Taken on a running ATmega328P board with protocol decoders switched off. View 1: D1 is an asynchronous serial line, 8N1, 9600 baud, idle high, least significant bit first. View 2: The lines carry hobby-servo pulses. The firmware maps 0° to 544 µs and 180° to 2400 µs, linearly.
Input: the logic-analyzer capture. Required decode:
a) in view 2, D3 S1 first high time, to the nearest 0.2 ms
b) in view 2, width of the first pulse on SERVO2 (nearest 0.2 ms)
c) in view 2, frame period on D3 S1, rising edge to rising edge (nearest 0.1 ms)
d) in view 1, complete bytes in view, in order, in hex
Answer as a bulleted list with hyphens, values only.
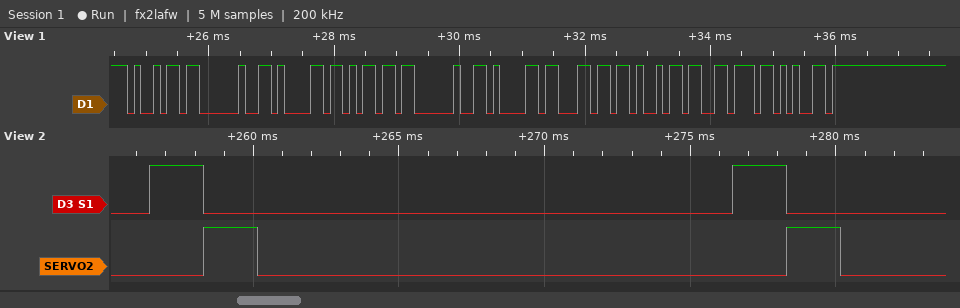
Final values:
- 1.8 ms
- 1.8 ms
- 20.0 ms
- 0x69 0x20 0x61 0x6D 0x20 0x61 0x6C 0x69 0x76 0x65
